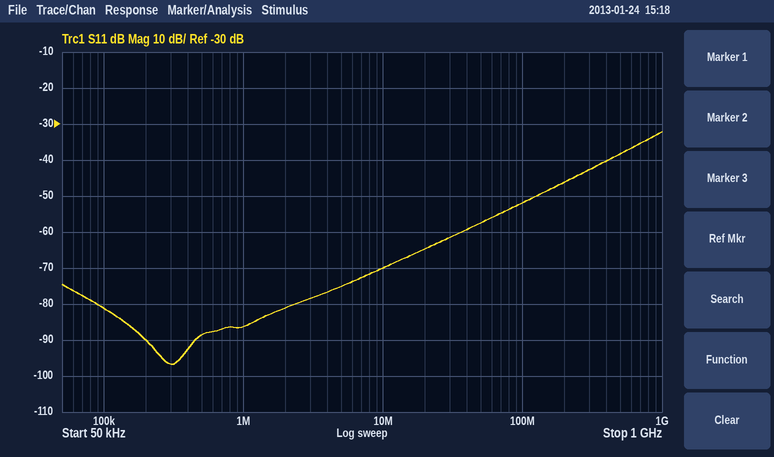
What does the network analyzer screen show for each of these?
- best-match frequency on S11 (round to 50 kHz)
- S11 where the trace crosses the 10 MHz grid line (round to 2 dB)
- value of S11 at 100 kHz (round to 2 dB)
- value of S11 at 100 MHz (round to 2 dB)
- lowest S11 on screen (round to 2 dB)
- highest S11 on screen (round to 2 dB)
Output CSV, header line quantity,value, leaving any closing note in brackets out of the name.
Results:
quantity,value
best-match frequency on S11,300 kHz
S11 where the trace crosses the 10 MHz grid line,-70 dB
value of S11 at 100 kHz,-82 dB
value of S11 at 100 MHz,-52 dB
lowest S11 on screen,-96 dB
highest S11 on screen,-32 dB
